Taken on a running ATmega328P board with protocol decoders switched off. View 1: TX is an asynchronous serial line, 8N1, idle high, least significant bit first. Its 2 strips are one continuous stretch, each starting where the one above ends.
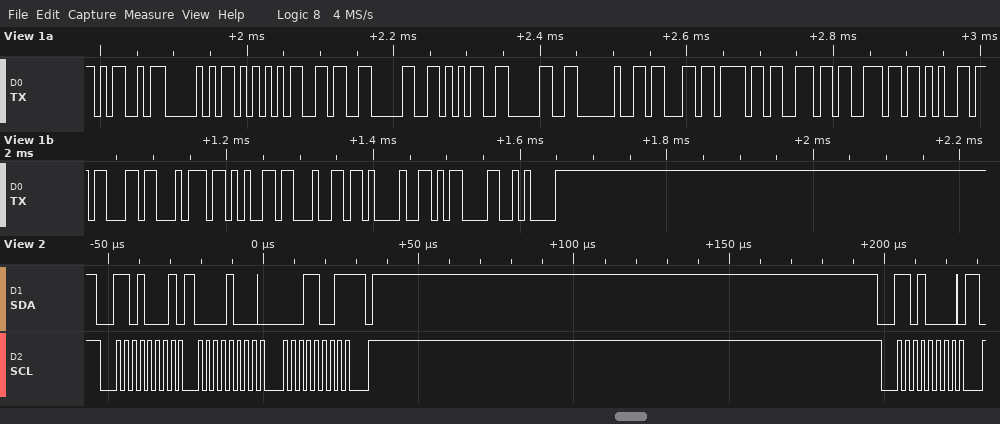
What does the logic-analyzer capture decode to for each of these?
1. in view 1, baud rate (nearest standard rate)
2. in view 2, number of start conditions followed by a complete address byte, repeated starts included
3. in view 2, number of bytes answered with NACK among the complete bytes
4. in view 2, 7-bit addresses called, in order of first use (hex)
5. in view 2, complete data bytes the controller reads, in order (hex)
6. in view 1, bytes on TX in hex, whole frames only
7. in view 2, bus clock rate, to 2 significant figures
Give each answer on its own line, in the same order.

115200 baud
2
1
0x68
08 19
0x4D 0x50 0x55 0x36 0x30 0x35 0x30 0x20 0x63 0x6F 0x6E 0x6E 0x65 0x63 0x74 0x65 0x64 0x21 0x0D 0x0A
400 kHz
